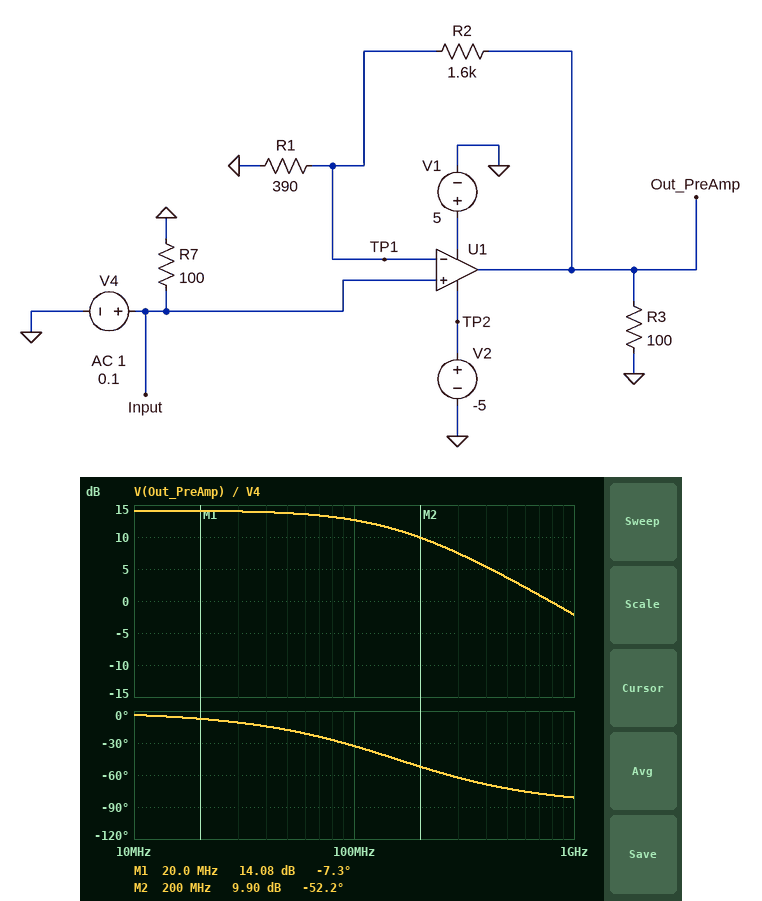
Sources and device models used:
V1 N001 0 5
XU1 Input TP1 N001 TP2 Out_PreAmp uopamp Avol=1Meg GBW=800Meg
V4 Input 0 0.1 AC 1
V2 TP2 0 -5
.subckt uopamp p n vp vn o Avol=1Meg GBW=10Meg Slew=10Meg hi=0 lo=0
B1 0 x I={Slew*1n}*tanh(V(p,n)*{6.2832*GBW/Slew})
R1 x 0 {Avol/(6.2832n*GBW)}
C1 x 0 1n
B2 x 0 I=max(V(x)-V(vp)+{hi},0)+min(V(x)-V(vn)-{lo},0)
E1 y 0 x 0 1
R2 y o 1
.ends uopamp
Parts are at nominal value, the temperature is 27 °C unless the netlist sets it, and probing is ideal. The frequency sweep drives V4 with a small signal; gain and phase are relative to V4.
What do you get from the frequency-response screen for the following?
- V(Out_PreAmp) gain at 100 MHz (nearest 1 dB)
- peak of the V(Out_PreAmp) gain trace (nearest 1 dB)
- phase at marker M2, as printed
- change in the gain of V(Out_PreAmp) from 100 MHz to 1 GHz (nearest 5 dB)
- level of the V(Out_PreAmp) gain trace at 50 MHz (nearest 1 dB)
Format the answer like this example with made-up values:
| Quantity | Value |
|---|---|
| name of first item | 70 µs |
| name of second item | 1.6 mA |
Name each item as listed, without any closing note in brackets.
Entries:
| Quantity | Value |
|---|---|
| V(Out_PreAmp) gain at 100 MHz | 13 dB |
| peak of the V(Out_PreAmp) gain trace | 14 dB |
| phase at marker M2, as printed | -52.2 deg |
| change in the gain of V(Out_PreAmp) from 100 MHz to 1 GHz | -15 dB |
| level of the V(Out_PreAmp) gain trace at 50 MHz | 14 dB |
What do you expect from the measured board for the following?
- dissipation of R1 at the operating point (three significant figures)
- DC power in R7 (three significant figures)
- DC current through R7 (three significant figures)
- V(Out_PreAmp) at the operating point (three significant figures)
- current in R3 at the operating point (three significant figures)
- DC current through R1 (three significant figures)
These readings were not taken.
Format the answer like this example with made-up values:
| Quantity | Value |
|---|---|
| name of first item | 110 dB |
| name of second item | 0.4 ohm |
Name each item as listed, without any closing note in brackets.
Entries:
| Quantity | Value |
|---|---|
| dissipation of R1 at the operating point | 25.6 µW |
| DC power in R7 | 100 µW |
| DC current through R7 | 1.00 mA |
| V(Out_PreAmp) at the operating point | 510 mV |
| current in R3 at the operating point | 5.10 mA |
| DC current through R1 | 256 µA |
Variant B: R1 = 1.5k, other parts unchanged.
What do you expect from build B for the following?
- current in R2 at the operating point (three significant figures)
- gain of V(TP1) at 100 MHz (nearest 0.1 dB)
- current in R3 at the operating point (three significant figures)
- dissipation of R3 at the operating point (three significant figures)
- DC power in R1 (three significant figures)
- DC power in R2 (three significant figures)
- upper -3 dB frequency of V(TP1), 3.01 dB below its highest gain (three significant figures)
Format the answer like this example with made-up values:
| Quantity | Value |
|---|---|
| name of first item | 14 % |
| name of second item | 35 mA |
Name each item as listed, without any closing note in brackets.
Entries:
| Quantity | Value |
|---|---|
| current in R2 at the operating point | 66.7 µA |
| gain of V(TP1) at 100 MHz | -0.3 dB |
| current in R3 at the operating point | 2.07 mA |
| dissipation of R3 at the operating point | 427 µW |
| DC power in R1 | 6.67 µW |
| DC power in R2 | 7.11 µW |
| upper -3 dB frequency of V(TP1), 3.01 dB below its highest gain | 383 MHz |
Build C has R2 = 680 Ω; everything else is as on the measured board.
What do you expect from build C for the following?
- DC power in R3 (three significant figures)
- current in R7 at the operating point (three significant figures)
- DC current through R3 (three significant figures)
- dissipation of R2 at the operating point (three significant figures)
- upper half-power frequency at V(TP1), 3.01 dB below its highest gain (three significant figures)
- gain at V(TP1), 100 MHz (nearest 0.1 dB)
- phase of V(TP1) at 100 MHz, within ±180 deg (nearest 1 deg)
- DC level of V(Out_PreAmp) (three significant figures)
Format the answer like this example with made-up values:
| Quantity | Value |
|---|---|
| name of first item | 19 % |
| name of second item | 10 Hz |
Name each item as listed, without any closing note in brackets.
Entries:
| Quantity | Value |
|---|---|
| DC power in R3 | 753 µW |
| current in R7 at the operating point | 1.00 mA |
| DC current through R3 | 2.74 mA |
| dissipation of R2 at the operating point | 44.7 µW |
| upper half-power frequency at V(TP1), 3.01 dB below its highest gain | 288 MHz |
| gain at V(TP1), 100 MHz | -0.5 dB |
| phase of V(TP1) at 100 MHz, within ±180 deg | -19 deg |
| DC level of V(Out_PreAmp) | 274 mV |
